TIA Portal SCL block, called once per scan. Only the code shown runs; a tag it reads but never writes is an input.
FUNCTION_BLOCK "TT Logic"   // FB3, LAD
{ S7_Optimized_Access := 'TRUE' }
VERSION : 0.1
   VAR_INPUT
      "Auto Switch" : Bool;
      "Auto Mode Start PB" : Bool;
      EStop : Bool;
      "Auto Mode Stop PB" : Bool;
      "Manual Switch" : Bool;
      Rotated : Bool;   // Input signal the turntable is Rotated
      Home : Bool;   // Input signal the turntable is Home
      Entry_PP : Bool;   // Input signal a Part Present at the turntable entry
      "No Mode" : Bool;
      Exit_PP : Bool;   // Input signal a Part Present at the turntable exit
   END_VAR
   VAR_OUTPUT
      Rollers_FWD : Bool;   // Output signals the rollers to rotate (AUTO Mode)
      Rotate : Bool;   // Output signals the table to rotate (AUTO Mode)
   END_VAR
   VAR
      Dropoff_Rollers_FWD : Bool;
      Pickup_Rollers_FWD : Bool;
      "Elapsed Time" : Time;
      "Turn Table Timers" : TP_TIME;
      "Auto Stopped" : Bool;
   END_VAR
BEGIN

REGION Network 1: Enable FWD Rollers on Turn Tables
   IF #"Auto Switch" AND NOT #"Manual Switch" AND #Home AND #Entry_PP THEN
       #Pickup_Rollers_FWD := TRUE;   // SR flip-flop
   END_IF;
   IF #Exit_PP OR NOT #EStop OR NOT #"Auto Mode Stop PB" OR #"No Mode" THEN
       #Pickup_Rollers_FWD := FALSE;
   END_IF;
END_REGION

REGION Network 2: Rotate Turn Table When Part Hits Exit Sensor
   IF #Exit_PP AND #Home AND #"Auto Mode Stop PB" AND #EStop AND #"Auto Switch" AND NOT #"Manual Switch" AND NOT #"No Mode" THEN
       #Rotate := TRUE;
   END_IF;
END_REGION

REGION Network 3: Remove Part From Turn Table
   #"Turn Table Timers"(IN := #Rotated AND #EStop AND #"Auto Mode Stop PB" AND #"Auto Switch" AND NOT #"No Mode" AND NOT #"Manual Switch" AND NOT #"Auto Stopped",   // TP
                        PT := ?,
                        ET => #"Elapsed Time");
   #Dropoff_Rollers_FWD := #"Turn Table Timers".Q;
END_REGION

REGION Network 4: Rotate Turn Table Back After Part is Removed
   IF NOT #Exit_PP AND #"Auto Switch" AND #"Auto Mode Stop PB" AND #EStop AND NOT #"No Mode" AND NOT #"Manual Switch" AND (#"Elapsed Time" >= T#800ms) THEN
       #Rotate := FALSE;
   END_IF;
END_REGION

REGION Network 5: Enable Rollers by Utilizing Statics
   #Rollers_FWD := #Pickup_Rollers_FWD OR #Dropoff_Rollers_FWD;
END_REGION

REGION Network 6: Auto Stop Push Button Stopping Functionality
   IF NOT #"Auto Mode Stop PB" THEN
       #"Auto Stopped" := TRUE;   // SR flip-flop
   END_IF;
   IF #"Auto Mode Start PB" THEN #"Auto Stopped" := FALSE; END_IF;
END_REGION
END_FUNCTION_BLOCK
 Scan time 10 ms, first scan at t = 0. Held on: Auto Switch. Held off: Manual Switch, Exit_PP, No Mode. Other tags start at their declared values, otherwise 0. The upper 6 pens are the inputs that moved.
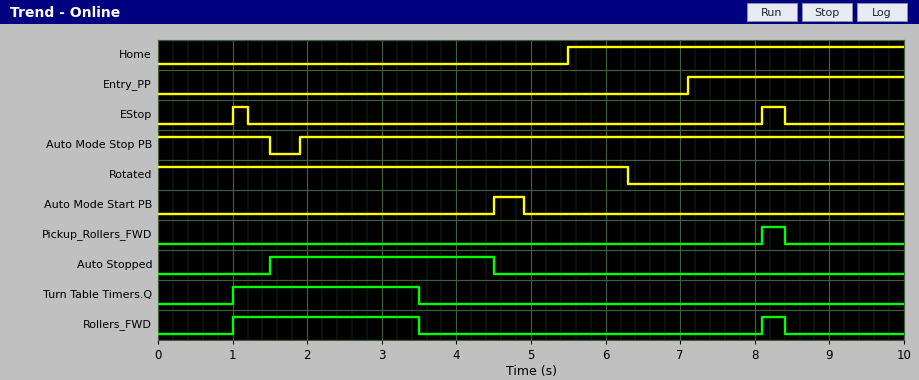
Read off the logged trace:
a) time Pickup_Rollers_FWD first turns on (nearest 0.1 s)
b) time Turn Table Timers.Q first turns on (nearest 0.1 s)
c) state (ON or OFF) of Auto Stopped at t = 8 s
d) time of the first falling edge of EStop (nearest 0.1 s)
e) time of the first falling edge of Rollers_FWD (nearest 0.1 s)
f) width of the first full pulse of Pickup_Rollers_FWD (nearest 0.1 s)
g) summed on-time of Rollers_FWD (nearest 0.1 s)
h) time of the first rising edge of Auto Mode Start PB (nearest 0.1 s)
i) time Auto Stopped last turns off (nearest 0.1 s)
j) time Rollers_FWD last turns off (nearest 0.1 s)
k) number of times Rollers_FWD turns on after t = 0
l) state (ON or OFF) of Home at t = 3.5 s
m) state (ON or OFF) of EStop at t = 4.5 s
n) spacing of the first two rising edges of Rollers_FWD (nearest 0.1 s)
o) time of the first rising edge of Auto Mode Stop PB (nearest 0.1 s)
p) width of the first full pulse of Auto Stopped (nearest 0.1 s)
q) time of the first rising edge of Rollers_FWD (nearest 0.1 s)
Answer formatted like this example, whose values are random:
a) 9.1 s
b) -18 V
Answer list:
a) 8.1 s
b) 1.0 s
c) OFF
d) 1.2 s
e) 3.5 s
f) 0.3 s
g) 2.8 s
h) 4.5 s
i) 4.5 s
j) 8.4 s
k) 2
l) OFF
m) OFF
n) 7.1 s
o) 1.9 s
p) 3.0 s
q) 1.0 s
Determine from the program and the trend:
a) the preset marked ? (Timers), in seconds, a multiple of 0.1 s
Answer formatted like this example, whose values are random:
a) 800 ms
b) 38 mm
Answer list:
a) 2.5 s
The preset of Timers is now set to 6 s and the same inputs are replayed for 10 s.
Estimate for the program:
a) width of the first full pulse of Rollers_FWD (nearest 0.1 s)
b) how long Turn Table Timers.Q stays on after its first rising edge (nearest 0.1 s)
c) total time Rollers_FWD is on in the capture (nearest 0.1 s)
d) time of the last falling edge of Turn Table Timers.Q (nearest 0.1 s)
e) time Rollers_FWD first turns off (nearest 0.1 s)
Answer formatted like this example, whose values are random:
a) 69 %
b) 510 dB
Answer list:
a) 6.0 s
b) 6.0 s
c) 6.3 s
d) 7.0 s
e) 7.0 s
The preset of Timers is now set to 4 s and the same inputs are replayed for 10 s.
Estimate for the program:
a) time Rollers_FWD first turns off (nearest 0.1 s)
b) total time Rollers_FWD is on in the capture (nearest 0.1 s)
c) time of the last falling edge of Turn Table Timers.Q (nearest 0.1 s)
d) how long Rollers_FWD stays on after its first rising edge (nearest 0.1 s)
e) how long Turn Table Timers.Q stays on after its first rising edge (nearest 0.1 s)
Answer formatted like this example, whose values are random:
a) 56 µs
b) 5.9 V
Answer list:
a) 5.0 s
b) 4.3 s
c) 5.0 s
d) 4.0 s
e) 4.0 s
